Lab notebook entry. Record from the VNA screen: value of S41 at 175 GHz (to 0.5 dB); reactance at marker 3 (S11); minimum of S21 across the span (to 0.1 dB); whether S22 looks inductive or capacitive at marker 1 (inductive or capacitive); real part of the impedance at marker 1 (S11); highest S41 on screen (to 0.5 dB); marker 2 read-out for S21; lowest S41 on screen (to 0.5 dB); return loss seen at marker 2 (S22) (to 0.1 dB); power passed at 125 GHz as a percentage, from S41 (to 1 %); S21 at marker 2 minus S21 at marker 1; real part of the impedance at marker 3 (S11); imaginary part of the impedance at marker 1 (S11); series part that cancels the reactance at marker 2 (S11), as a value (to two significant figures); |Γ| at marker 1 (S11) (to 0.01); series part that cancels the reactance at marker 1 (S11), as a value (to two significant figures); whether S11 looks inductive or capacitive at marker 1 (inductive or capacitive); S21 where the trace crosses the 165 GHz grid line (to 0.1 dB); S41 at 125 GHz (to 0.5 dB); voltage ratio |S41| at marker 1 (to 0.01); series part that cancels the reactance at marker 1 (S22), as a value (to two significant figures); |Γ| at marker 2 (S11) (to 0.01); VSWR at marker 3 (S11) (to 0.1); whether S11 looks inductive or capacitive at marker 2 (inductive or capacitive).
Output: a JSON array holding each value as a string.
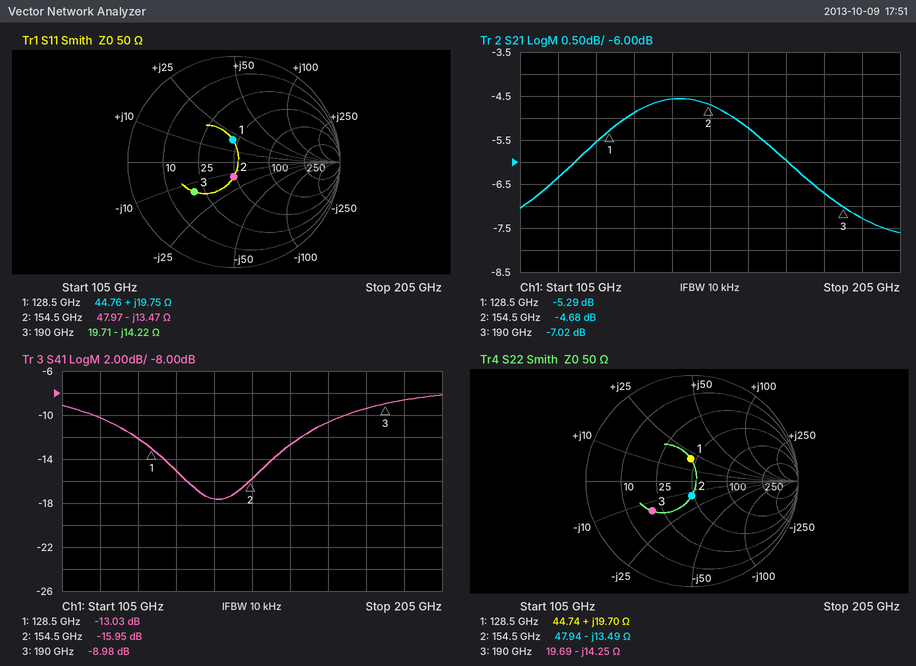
["-10.5 dB", "-14.22 Ω", "-7.6 dB", "inductive", "44.76 Ω", "-8.0 dB", "-4.68 dB", "-17.5 dB", "17.2 dB", "6 %", "0.61 dB", "19.71 Ω", "+19.75 Ω", "14 pH", "0.21", "63 fF", "inductive", "-5.2 dB", "-12.0 dB", "0.22", "63 fF", "0.14", "2.8", "capacitive"]
